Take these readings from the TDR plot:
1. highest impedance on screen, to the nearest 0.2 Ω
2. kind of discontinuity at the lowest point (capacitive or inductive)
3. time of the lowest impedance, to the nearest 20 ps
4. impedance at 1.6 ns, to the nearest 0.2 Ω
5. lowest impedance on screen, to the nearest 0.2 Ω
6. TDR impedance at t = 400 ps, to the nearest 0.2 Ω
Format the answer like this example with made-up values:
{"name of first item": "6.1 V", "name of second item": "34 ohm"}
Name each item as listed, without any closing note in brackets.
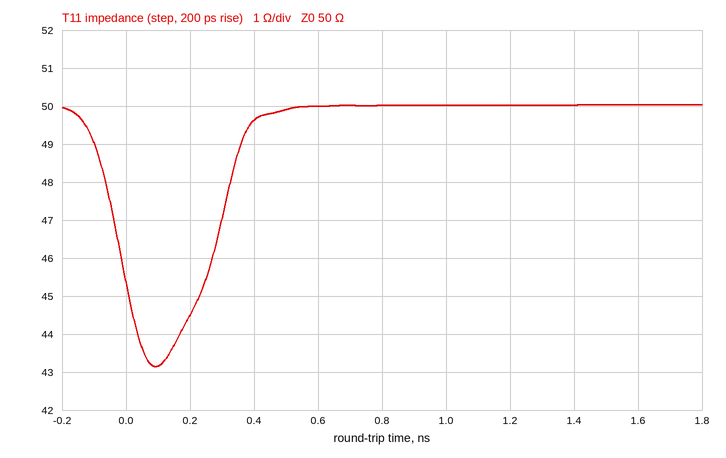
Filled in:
{"highest impedance on screen, to the nearest 0.2 Ω": "50.0 Ω", "kind of discontinuity at the lowest point": "capacitive", "time of the lowest impedance, to the nearest 20 ps": "100 ps", "impedance at 1.6 ns, to the nearest 0.2 Ω": "50.0 Ω", "lowest impedance on screen, to the nearest 0.2 Ω": "43.2 Ω", "TDR impedance at t = 400 ps, to the nearest 0.2 Ω": "49.6 Ω"}
